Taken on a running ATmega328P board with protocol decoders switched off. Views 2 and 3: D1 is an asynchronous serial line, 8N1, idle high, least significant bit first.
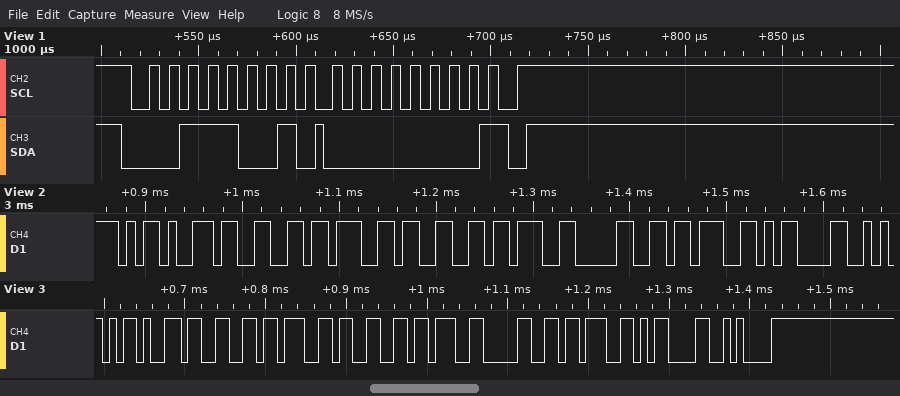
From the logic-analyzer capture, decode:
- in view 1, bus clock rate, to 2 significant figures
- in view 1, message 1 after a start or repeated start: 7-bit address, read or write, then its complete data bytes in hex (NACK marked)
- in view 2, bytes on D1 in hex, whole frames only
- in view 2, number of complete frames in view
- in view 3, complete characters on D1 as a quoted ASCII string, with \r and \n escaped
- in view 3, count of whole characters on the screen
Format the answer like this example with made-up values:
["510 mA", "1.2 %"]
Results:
["100 kHz", "0x1C read: 00 NACK", "2D 33 3B 33 3B 30 3B 0D", "8", "\"-3;3;0;\\r\\n\"", "9"]
